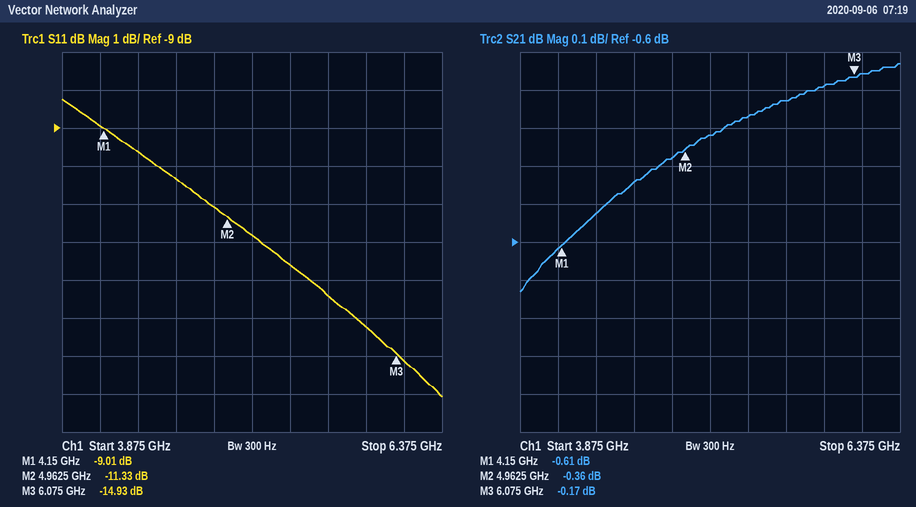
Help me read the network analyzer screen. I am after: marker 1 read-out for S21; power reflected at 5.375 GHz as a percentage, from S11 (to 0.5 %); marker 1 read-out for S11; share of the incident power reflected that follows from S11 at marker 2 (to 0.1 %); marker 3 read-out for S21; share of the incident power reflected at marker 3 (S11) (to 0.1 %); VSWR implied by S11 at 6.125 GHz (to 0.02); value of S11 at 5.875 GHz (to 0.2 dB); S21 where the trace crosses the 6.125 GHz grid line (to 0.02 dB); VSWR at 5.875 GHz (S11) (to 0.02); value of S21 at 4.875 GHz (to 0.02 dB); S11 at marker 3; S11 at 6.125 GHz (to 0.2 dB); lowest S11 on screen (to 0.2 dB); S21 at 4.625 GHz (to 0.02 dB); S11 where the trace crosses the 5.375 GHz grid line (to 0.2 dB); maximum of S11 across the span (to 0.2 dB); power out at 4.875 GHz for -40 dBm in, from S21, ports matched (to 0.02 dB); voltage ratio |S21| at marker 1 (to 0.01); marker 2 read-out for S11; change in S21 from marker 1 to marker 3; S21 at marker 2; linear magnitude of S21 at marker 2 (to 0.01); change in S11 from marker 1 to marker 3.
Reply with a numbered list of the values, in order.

1. -0.61 dB
2. 5.5 %
3. -9.01 dB
4. 7.4 %
5. -0.17 dB
6. 3.2 %
7. 1.42
8. -14.2 dB
9. -0.16 dB
10. 1.48
11. -0.38 dB
12. -14.93 dB
13. -15.2 dB
14. -16.0 dB
15. -0.44 dB
16. -12.6 dB
17. -8.2 dB
18. -40.38 dBm
19. 0.93
20. -11.33 dB
21. 0.44 dB
22. -0.36 dB
23. 0.96
24. -5.92 dB
